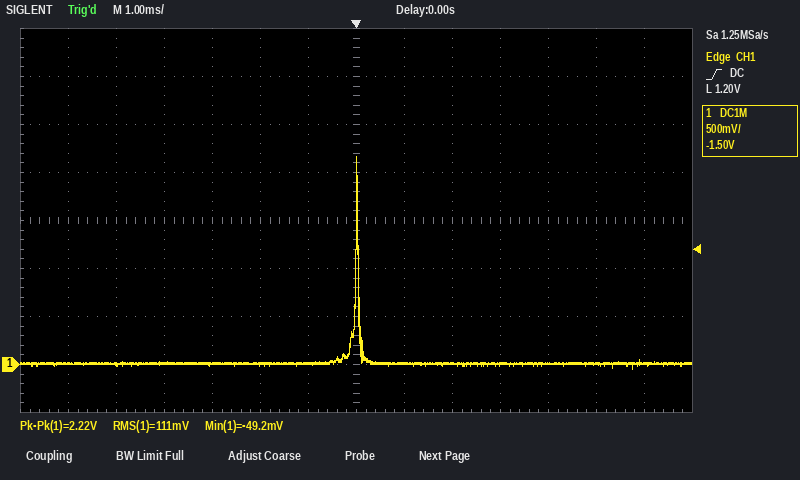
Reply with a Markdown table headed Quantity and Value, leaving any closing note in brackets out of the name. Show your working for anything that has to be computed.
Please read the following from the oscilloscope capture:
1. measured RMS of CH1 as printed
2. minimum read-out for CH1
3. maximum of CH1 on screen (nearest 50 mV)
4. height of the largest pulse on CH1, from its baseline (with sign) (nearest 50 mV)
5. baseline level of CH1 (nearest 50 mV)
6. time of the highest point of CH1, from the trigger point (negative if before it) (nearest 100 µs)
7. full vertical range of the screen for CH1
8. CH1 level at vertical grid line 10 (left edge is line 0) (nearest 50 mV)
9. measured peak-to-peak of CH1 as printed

| Quantity | Value |
|---|---|
| measured RMS of CH1 as printed | 111 mV |
| minimum read-out for CH1 | -49.2 mV |
| maximum of CH1 on screen | 2.15 V |
| height of the largest pulse on CH1, from its baseline (with sign) | 2.15 V − (0 mV) = +2.15 V |
| baseline level of CH1 | 0 mV |
| time of the highest point of CH1, from the trigger point (negative if before it) | 0.0 ms |
| full vertical range of the screen for CH1 | 4 V |
| CH1 level at vertical grid line 10 (left edge is line 0) | 0 mV |
| measured peak-to-peak of CH1 as printed | 2.22 V |
